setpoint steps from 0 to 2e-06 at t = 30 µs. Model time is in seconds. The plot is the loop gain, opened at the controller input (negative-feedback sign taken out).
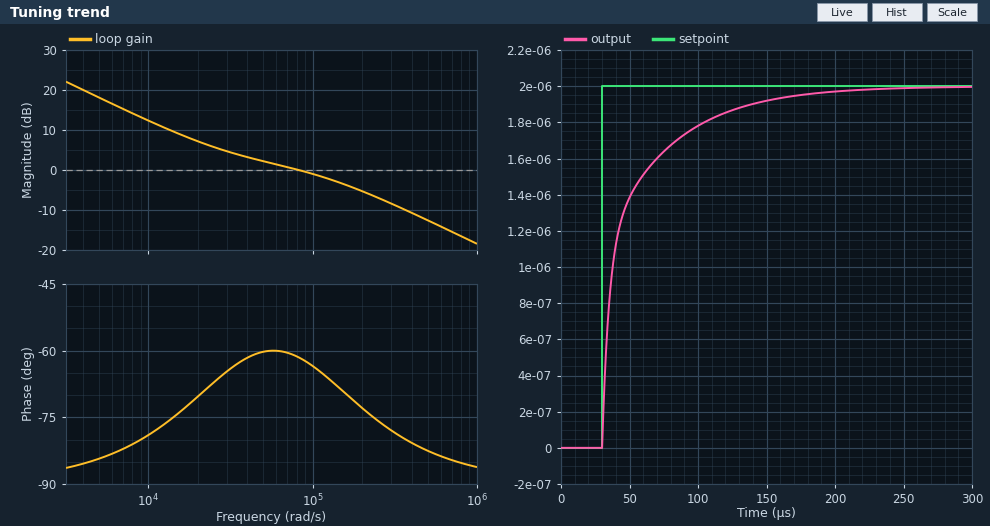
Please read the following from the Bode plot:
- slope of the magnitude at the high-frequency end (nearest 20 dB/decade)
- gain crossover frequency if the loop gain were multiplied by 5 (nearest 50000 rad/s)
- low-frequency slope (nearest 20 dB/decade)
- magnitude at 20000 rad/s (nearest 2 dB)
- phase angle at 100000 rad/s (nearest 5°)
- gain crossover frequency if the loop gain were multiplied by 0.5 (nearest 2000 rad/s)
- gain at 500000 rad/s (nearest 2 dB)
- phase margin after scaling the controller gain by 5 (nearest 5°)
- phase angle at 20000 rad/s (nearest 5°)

-20 dB/decade
600000 rad/s
-20 dB/decade
8 dB
-65°
24000 rad/s
-12 dB
95°
-70°
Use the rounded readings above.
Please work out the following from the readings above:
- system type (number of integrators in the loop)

1
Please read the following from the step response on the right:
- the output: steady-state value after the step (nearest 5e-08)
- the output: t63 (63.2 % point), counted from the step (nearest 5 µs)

0.00000200
15 µs
